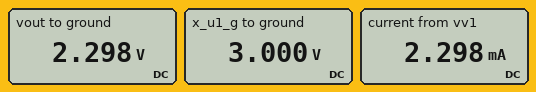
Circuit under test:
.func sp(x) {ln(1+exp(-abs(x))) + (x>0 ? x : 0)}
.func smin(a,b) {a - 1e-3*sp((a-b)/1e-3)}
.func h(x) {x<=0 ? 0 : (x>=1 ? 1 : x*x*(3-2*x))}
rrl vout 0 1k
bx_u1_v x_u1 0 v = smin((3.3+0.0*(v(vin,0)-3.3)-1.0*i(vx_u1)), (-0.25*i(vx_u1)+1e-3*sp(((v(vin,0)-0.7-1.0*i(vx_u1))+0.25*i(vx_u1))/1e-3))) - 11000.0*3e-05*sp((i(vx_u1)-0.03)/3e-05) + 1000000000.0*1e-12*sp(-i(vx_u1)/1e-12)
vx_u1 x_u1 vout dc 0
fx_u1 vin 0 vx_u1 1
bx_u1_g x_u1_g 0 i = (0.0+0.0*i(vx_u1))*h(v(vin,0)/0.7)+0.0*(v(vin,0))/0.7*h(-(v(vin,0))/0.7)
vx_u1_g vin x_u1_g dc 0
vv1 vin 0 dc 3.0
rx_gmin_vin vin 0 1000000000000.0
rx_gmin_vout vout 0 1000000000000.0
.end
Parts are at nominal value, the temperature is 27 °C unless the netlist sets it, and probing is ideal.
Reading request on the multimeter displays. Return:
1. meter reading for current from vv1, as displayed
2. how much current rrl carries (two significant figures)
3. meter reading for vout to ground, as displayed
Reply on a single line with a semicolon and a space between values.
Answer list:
2.298 mA; 2.3 mA; 2.298 V
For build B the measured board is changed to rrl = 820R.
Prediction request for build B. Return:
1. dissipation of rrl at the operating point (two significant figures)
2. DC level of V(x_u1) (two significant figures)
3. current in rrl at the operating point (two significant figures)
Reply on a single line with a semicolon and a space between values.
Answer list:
6.4 mW; 2.3 V; 2.8 mA
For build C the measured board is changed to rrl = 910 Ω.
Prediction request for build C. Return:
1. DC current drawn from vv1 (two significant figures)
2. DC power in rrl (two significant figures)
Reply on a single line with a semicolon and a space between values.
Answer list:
2.5 mA; 5.8 mW
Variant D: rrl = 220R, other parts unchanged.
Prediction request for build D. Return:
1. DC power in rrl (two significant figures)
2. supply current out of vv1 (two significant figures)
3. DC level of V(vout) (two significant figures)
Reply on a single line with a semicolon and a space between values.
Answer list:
24 mW; 10 mA; 2.3 V
